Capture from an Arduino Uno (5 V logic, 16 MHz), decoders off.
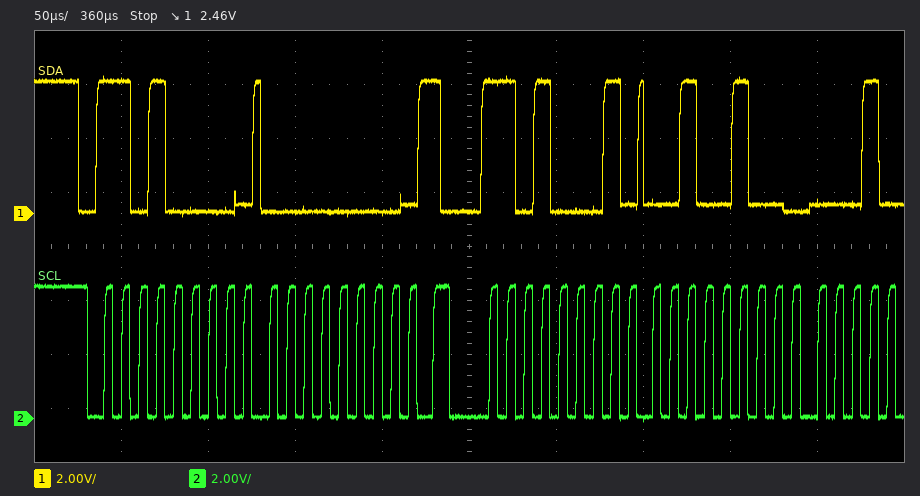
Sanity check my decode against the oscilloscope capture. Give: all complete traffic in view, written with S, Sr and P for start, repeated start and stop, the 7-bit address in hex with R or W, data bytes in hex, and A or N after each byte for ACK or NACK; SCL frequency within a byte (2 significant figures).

S 68W A 00 A Sr 68R A 24 A
100 kHz
